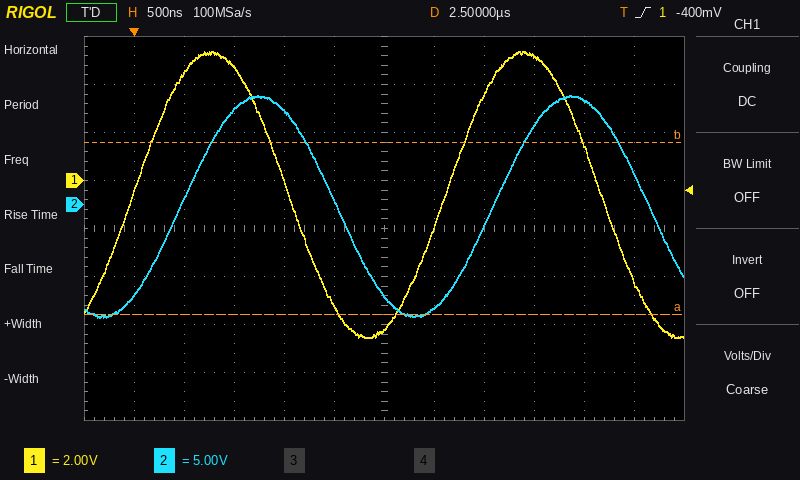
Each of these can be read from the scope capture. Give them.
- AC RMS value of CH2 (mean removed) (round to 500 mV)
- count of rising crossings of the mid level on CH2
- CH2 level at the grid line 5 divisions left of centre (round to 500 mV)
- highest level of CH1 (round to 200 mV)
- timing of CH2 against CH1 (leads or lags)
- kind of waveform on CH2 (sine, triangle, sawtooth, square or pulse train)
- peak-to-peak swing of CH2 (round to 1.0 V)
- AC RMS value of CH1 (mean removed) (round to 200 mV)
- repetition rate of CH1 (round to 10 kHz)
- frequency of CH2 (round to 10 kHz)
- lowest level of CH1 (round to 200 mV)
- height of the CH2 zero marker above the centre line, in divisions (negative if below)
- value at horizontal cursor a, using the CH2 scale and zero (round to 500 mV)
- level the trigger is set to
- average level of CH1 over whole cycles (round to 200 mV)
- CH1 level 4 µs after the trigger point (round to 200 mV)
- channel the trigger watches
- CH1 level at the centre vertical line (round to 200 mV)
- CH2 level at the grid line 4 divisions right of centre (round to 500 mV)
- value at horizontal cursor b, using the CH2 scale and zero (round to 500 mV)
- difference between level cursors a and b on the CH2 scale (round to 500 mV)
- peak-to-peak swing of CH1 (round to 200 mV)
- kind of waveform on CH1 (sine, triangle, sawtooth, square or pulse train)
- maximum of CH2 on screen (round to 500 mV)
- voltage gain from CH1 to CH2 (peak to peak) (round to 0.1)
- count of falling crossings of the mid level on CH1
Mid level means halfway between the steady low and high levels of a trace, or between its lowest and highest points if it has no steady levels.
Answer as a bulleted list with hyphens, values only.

- 8.0 V
- 2
- -9.5 V
- 5.4 V
- lags
- sine
- 23.0 V
- 4.2 V
- 320 kHz
- 320 kHz
- -6.6 V
- +0.5 div
- -11.5 V
- -400 mV
- -600 mV
- 5.2 V
- CH1
- -6.2 V
- 11.0 V
- 6.5 V
- 18.0 V
- 12.0 V
- sine
- 11.5 V
- 1.9
- 2
